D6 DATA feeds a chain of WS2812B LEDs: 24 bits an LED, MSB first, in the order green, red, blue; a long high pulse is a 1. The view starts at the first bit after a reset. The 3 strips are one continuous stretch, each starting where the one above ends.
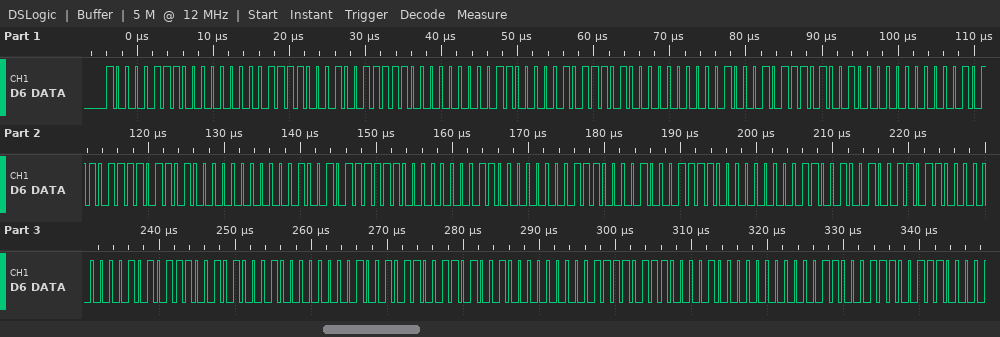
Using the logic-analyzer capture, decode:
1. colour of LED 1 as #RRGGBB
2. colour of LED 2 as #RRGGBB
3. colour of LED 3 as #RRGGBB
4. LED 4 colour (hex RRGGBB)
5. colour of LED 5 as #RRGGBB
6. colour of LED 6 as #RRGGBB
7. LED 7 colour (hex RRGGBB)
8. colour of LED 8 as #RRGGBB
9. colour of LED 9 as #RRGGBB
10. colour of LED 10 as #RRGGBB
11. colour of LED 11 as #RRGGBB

#008778
#009F60
#00BA45
#00D22D
#00ED12
#03FC00
#1EE100
#36C900
#51AE00
#699600
#847B00
